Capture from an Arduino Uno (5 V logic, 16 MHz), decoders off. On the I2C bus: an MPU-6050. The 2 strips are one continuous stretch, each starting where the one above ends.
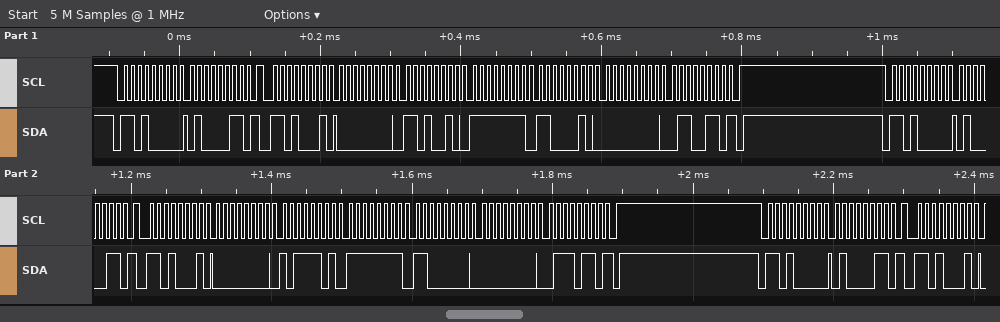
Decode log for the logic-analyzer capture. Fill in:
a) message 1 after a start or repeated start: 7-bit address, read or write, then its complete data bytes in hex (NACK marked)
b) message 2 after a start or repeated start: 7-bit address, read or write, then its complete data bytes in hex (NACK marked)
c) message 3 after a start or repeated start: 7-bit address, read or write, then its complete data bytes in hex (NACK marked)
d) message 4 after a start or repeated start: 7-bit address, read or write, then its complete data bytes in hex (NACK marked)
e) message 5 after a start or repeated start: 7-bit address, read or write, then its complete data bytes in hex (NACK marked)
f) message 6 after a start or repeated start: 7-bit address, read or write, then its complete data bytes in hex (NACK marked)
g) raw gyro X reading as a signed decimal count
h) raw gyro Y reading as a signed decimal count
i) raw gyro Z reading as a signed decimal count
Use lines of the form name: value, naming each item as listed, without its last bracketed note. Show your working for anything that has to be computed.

message 1 after a start or repeated start: 7-bit address, read or write, then its complete data bytes in hex: 0x68 write: 43
message 2 after a start or repeated start: 7-bit address, read or write, then its complete data bytes in hex: 0x68 read: 00 D2 FF C2 00 66 NACK
message 3 after a start or repeated start: 7-bit address, read or write, then its complete data bytes in hex: 0x68 write: 43
message 4 after a start or repeated start: 7-bit address, read or write, then its complete data bytes in hex: 0x68 read: 00 BD FF C0 00 76 NACK
message 5 after a start or repeated start: 7-bit address, read or write, then its complete data bytes in hex: 0x68 write: 43
message 6 after a start or repeated start: 7-bit address, read or write, then its complete data bytes in hex: 0x68 read
raw gyro X reading as a signed decimal count: 0x00D2 = 210
raw gyro Y reading as a signed decimal count: 0xFFC2 = -62
raw gyro Z reading as a signed decimal count: 0x0066 = 102
